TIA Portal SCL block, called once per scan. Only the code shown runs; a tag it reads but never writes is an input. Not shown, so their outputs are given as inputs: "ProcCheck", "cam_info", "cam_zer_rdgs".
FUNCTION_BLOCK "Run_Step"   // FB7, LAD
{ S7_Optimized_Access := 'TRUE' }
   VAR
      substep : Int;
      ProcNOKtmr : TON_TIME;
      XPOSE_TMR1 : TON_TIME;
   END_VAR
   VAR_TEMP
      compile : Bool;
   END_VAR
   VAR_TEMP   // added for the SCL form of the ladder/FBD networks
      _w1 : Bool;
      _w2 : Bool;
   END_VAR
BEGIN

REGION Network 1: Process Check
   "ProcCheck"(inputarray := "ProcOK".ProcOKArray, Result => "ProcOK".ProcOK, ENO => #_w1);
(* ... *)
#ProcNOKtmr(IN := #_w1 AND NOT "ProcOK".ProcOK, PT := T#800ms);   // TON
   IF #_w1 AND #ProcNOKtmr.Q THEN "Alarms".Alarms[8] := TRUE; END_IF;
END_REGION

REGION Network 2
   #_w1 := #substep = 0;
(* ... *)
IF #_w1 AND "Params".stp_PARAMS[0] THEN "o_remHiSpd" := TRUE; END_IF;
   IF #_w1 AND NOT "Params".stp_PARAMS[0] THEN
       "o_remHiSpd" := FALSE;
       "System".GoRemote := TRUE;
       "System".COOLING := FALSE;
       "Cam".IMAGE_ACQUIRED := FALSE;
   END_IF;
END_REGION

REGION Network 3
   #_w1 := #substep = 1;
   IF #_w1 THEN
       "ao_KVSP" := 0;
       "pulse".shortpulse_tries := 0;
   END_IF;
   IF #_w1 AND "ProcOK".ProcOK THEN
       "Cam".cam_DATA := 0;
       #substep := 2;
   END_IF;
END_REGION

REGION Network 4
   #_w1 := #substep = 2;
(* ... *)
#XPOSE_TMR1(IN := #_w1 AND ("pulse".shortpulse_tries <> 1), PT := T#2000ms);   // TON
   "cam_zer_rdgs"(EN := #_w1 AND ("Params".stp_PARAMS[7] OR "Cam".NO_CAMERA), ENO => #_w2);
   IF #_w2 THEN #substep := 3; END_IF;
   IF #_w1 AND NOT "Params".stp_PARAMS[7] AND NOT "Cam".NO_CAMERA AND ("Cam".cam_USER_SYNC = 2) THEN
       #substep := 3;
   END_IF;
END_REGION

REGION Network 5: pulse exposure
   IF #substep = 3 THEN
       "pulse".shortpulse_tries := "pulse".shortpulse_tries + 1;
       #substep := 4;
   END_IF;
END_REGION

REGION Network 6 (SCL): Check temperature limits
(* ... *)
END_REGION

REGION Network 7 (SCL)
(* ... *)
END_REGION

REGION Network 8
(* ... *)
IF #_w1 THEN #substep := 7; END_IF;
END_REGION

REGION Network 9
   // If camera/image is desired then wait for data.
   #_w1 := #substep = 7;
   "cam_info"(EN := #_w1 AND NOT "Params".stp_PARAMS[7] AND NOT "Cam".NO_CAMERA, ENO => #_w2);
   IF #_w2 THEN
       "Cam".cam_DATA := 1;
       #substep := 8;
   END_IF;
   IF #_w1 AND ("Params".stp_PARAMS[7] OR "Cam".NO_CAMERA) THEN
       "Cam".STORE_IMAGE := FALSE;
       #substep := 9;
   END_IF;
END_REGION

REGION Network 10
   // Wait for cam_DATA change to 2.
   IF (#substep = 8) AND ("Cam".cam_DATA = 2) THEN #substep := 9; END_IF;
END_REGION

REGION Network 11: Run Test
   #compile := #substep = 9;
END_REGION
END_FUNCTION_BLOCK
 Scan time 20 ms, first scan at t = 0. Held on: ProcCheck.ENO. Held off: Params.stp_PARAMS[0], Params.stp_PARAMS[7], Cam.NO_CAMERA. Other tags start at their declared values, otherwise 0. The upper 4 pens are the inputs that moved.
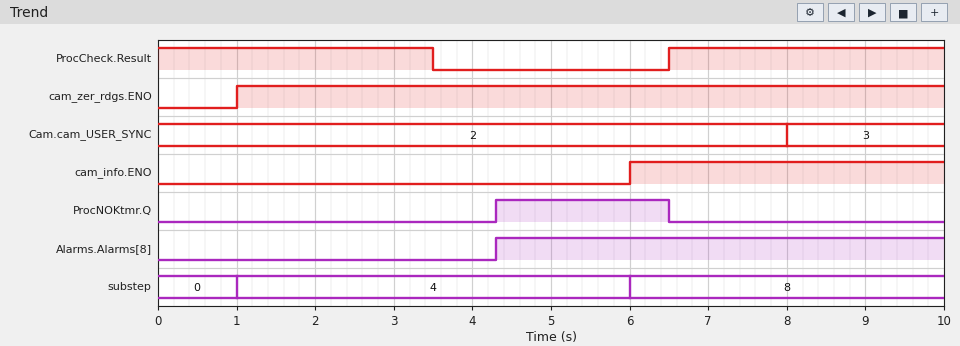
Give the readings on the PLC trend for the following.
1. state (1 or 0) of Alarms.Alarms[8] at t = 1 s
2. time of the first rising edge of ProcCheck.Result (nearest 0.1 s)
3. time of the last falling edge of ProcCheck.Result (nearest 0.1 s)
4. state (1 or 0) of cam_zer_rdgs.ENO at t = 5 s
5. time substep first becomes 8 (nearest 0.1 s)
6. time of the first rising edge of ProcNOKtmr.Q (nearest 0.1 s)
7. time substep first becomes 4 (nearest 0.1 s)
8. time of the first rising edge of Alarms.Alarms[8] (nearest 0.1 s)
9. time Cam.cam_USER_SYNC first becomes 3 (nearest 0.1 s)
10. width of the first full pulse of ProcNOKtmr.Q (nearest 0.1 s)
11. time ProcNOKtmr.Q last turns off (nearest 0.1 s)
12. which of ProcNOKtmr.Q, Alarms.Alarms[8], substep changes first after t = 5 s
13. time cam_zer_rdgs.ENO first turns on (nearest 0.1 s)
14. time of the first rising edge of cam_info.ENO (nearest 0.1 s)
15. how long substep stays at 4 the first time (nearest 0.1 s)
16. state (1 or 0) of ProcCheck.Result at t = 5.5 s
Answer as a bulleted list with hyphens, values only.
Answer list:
- 0
- 6.5 s
- 3.5 s
- 1
- 6.0 s
- 4.3 s
- 1.0 s
- 4.3 s
- 8.0 s
- 2.2 s
- 6.5 s
- substep
- 1.0 s
- 6.0 s
- 5.0 s
- 0
